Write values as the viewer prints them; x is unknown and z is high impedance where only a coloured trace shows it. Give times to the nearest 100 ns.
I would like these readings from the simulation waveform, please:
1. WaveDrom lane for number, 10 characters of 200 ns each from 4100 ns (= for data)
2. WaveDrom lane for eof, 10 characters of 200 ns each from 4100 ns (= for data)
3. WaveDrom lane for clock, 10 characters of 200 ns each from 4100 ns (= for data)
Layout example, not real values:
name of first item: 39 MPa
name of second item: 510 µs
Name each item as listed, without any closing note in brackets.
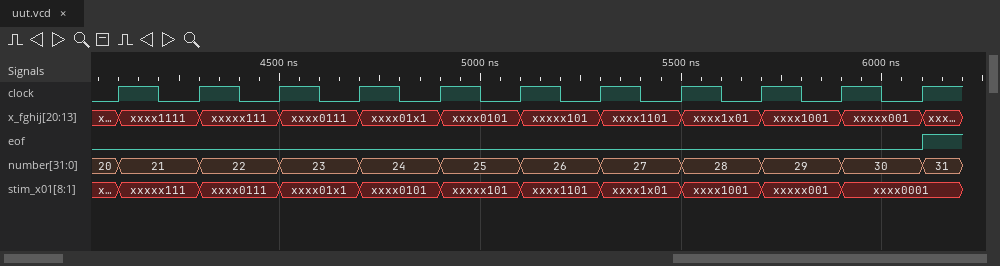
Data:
WaveDrom lane for number, 10 characters of 200 ns each from 4100 ns: {name: 'number', wave: '==========', data: '21 22 23 24 25 26 27 28 29 30'}
WaveDrom lane for eof, 10 characters of 200 ns each from 4100 ns: {name: 'eof', wave: '0.........'}
WaveDrom lane for clock, 10 characters of 200 ns each from 4100 ns: {name: 'clock', wave: 'p.........'}
